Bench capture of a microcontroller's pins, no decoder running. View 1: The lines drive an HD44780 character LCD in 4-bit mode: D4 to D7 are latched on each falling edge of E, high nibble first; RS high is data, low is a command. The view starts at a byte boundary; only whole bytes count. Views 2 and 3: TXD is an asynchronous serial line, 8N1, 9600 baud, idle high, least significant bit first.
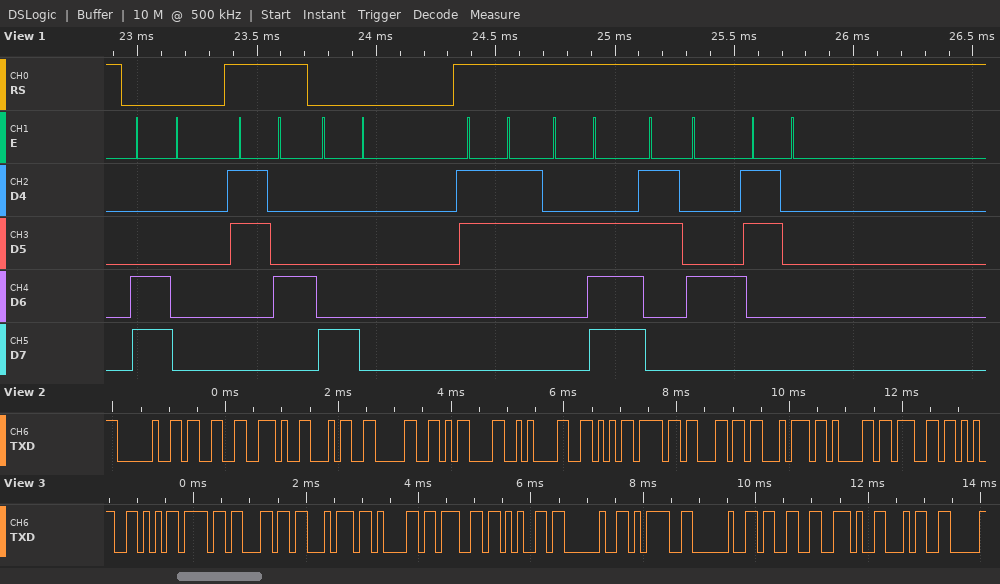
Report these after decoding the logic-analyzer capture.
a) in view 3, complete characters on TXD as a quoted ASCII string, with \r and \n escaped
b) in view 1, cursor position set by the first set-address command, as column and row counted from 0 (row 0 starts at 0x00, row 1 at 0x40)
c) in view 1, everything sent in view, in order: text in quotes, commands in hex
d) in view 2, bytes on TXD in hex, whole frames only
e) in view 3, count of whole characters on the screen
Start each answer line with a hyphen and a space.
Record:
- "Voltage = 3.4"
- column 0, row 1
- 0xC0 "4" 0x80 "3.40"
- 20 33 2E 34 30 0D 0A 56 6F 6C 74 61 67
- 13
